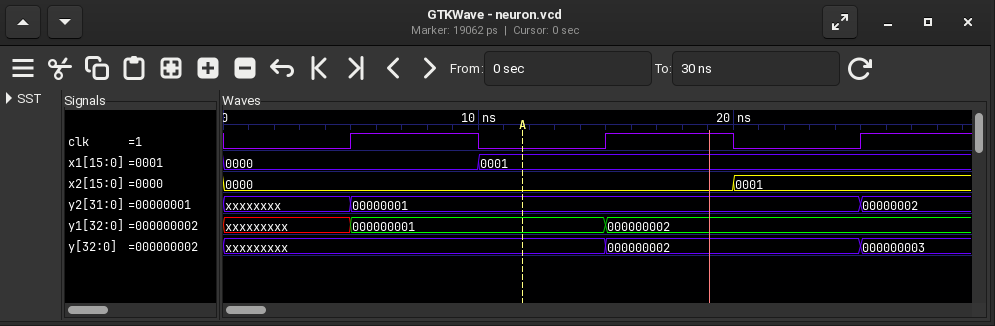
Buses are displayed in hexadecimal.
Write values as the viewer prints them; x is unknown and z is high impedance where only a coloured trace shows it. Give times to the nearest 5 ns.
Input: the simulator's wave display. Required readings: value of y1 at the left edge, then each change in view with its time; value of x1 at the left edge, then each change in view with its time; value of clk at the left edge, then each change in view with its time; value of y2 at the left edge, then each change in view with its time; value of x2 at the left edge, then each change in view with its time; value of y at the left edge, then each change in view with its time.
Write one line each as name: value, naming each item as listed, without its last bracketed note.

value of y1 at the left edge, then each change in view with its time: xxxxxxxxx, 000000001 at 5 ns, 000000002 at 15 ns
value of x1 at the left edge, then each change in view with its time: 0000, 0001 at 10 ns
value of clk at the left edge, then each change in view with its time: 0, 1 at 5 ns, 0 at 10 ns, 1 at 15 ns, 0 at 20 ns, 1 at 25 ns
value of y2 at the left edge, then each change in view with its time: xxxxxxxx, 00000001 at 5 ns, 00000002 at 25 ns
value of x2 at the left edge, then each change in view with its time: 0000, 0001 at 20 ns
value of y at the left edge, then each change in view with its time: xxxxxxxxx, 000000002 at 15 ns, 000000003 at 25 ns
